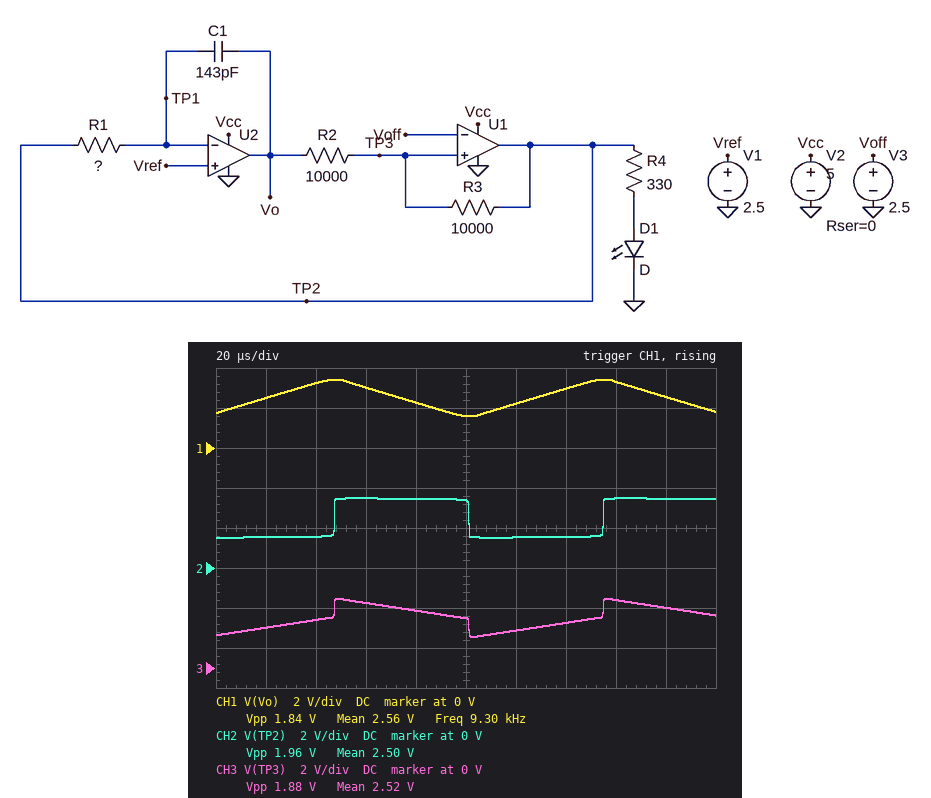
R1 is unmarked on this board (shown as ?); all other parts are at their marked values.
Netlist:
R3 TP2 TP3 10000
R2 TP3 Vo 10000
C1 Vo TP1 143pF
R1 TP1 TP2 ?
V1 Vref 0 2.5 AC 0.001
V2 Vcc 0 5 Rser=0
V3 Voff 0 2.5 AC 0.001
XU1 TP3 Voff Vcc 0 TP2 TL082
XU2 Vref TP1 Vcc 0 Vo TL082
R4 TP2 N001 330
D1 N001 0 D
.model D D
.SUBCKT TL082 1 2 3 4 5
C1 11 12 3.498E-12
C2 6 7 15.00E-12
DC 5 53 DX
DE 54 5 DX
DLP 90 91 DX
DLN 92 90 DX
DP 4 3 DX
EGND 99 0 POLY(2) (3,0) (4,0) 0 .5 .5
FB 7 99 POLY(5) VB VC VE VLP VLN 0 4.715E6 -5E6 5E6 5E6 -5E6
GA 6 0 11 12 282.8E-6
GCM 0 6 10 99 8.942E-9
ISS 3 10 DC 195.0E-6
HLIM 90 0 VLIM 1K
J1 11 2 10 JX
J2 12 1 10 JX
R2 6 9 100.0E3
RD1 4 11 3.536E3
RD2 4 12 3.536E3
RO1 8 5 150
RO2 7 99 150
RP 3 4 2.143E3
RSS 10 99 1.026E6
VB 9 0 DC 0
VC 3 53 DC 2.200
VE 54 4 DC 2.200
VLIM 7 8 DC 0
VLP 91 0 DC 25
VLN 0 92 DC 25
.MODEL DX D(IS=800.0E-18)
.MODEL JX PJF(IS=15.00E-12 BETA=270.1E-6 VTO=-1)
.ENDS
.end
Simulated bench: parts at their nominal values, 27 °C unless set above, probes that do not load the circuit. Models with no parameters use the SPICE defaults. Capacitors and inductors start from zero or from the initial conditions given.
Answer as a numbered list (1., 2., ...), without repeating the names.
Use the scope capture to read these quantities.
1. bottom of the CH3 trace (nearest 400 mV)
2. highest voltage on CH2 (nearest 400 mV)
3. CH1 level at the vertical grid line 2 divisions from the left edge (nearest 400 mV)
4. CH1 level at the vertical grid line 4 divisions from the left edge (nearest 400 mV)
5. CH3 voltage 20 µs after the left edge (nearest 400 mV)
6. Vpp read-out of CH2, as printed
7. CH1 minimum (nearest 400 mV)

1. 1.6 V
2. 3.6 V
3. 3.2 V
4. 2.4 V
5. 2.0 V
6. 1.96 V
7. 1.6 V
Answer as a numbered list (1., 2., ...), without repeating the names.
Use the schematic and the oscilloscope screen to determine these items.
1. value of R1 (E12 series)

1. 180 kΩ
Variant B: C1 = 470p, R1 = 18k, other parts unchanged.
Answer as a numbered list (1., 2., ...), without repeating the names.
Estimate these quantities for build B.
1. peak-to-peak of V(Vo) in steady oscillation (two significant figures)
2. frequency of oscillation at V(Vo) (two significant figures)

1. 1.9 V
2. 23 kHz
